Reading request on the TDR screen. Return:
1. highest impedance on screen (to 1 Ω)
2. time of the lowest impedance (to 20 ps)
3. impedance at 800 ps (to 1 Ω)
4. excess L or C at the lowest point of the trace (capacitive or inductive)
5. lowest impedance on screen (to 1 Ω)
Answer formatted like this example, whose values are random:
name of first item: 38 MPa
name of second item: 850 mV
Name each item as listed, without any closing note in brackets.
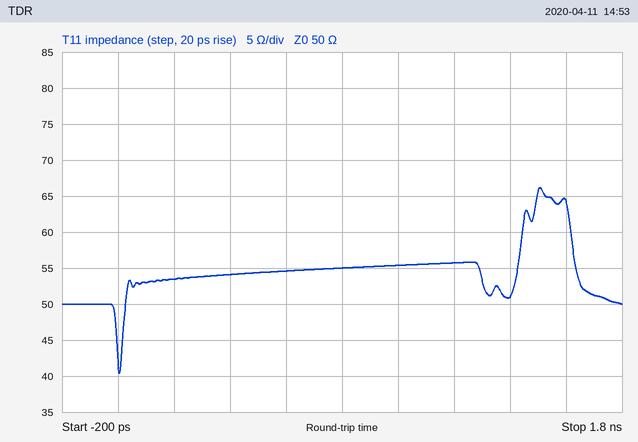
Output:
highest impedance on screen: 66 Ω
time of the lowest impedance: 0 ps
impedance at 800 ps: 55 Ω
excess L or C at the lowest point of the trace: capacitive
lowest impedance on screen: 40 Ω
